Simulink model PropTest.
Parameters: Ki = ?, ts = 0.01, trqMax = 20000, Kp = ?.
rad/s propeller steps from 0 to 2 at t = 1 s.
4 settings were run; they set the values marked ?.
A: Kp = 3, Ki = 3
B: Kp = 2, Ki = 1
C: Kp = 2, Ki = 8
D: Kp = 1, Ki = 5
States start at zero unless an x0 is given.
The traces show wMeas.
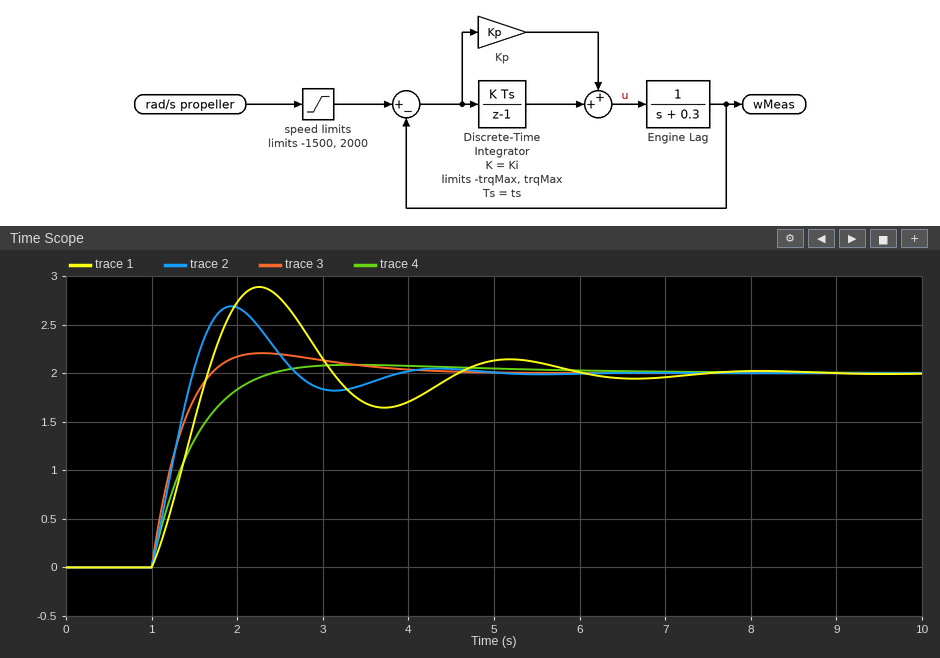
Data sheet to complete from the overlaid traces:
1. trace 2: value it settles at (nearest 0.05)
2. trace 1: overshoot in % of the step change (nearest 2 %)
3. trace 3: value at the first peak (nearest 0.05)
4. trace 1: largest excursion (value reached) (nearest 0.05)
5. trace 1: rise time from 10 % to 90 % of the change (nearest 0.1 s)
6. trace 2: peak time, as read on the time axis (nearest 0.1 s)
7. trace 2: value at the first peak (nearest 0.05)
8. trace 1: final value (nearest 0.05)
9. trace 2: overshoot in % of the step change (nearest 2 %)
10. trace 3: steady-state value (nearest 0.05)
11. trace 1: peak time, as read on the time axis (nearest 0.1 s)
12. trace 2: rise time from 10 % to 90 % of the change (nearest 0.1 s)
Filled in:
2.00
44 %
2.20
2.90
0.5 s
1.9 s
2.70
2.00
34 %
2.00
2.3 s
0.4 s
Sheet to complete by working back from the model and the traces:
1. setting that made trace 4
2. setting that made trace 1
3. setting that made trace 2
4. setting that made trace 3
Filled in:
B
D
C
A
